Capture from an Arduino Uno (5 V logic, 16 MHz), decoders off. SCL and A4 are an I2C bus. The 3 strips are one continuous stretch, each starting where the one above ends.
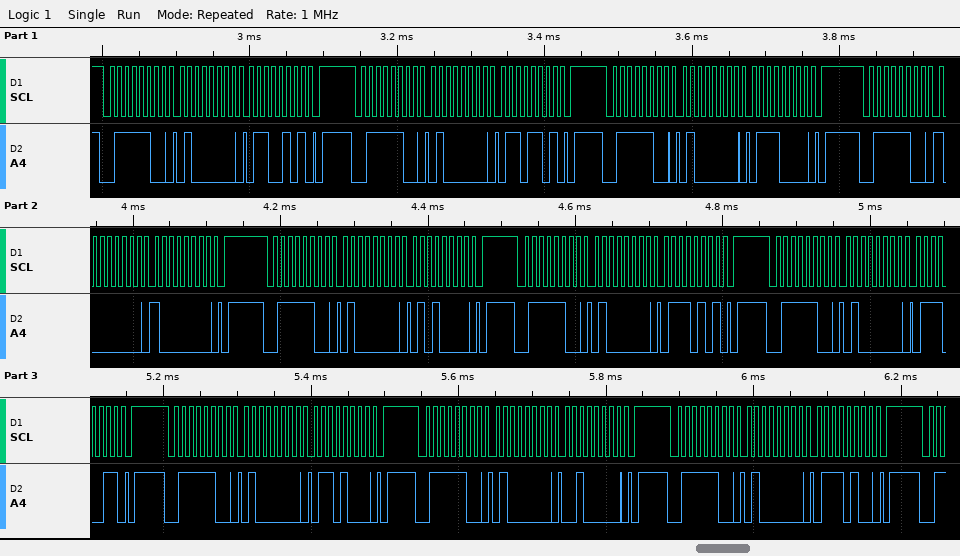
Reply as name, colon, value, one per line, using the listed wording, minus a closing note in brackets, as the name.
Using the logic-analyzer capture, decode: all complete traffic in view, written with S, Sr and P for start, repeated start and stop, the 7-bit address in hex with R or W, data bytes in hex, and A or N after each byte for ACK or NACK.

all complete traffic in view, written with S, Sr and P for start, repeated start and stop, the 7-bit address in hex with R or W, data bytes in hex, and A or N after each byte for ACK or NACK: S 3EW A 40 A 65 A P S 3EW A 40 A 6D A P S 3EW A 40 A 70 A P S 3EW A 80 A 80 A P S 3EW A 40 A 50 A P S 3EW A 40 A 75 A P S 3EW A 40 A 73 A P S 3EW A 40 A 68 A P S 3EW A 40 A 20 A P S 3EW A 40 A 74 A P
